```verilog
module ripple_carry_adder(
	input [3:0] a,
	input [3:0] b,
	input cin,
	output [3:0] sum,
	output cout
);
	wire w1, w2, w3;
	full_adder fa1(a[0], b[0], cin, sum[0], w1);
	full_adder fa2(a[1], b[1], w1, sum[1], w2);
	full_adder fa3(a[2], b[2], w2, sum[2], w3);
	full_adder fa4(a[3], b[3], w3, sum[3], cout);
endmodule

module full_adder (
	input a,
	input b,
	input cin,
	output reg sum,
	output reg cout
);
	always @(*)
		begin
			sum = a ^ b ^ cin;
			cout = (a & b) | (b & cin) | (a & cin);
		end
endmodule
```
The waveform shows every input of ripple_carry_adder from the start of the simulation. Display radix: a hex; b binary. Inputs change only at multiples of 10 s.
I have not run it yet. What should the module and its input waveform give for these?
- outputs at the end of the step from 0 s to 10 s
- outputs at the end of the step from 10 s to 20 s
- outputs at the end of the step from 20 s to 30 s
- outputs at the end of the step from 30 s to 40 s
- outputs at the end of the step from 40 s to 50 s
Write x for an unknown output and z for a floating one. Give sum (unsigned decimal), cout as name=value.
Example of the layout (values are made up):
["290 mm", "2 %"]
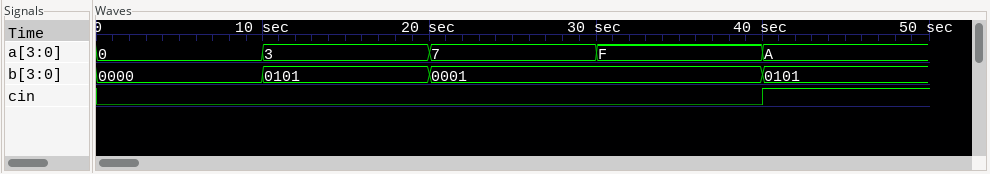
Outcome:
["sum=0, cout=0", "sum=8, cout=0", "sum=8, cout=0", "sum=0, cout=1", "sum=0, cout=1"]
